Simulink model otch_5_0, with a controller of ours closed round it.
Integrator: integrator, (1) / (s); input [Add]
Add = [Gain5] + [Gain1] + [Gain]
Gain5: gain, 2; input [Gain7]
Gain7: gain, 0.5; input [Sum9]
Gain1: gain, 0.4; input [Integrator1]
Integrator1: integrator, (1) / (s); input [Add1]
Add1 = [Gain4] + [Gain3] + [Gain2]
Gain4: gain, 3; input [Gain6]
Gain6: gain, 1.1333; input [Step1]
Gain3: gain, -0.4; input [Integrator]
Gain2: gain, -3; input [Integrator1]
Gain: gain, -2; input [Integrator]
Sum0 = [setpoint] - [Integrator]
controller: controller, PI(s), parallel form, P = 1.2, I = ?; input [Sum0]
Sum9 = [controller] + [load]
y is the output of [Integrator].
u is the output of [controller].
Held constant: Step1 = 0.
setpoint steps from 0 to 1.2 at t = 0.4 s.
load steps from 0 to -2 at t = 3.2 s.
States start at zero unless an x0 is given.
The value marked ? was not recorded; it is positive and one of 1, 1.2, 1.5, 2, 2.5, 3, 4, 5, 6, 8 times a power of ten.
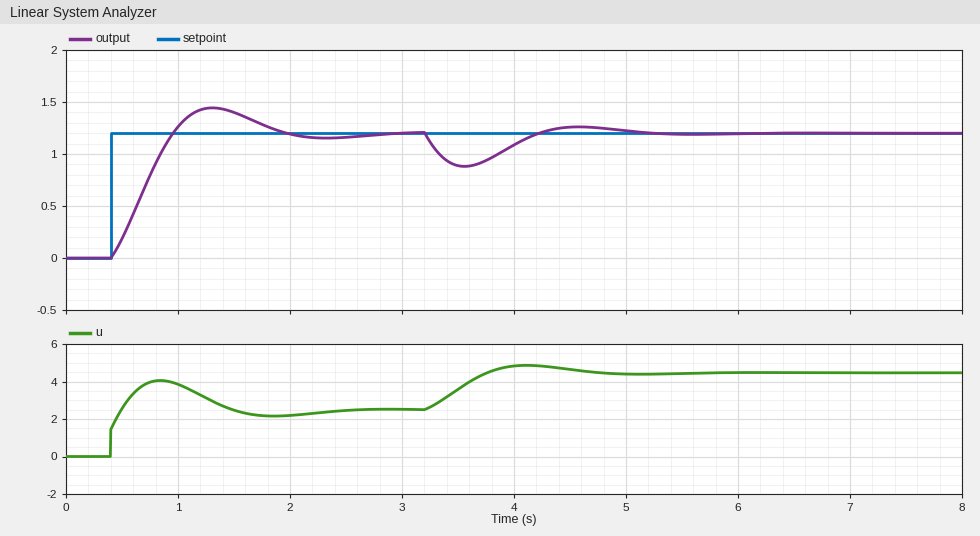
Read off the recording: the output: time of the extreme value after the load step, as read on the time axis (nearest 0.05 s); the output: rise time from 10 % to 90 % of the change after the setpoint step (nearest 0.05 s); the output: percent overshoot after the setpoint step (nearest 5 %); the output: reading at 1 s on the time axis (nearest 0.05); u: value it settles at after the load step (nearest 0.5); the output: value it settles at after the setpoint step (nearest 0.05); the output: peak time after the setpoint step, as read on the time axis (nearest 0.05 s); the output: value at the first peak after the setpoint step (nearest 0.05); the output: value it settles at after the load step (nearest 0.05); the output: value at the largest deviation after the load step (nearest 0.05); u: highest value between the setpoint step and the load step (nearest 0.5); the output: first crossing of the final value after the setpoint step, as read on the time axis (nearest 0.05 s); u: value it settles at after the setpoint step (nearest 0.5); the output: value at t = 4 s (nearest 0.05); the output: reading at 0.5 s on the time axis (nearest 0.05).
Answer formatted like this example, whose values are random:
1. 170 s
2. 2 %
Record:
1. 3.55 s
2. 0.40 s
3. 20 %
4. 1.25
5. 4.5
6. 1.20
7. 1.30 s
8. 1.45
9. 1.20
10. 0.90
11. 4.0
12. 0.95 s
13. 2.5
14. 1.10
15. 0.20
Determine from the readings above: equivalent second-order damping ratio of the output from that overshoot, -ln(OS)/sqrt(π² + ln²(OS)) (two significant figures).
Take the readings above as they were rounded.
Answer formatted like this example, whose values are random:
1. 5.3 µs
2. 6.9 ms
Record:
1. 0.46
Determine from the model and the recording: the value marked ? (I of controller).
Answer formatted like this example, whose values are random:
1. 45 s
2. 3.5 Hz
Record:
1. 12
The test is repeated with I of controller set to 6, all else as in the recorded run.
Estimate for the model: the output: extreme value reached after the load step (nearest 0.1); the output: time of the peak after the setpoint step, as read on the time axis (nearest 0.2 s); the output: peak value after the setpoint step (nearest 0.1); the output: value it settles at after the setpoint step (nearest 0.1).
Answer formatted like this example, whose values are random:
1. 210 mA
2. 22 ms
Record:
1. 0.8
2. 1.8 s
3. 1.3
4. 1.2
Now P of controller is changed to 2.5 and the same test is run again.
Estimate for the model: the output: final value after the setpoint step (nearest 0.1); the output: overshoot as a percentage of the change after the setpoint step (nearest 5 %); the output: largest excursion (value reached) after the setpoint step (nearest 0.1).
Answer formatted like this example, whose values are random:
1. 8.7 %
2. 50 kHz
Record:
1. 1.2
2. 10 %
3. 1.3
